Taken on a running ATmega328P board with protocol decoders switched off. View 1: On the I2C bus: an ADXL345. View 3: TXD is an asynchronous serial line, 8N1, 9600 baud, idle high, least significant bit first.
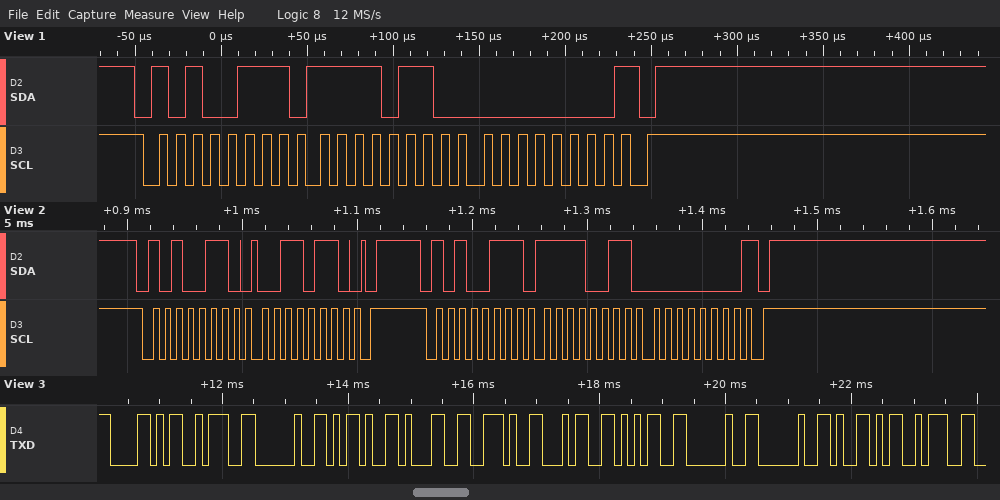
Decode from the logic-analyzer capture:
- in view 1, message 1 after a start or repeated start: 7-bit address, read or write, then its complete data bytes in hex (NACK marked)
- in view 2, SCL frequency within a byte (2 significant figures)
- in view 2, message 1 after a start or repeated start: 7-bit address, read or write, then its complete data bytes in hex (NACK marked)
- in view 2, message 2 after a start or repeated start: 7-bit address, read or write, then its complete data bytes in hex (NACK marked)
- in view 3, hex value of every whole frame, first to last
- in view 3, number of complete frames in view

0x53 read: F6 00 NACK
100 kHz
0x53 write: 36
0x53 read: F3 00 NACK
58 3A 20 2D 31 2E 34 35 20 20 59 3A
12
